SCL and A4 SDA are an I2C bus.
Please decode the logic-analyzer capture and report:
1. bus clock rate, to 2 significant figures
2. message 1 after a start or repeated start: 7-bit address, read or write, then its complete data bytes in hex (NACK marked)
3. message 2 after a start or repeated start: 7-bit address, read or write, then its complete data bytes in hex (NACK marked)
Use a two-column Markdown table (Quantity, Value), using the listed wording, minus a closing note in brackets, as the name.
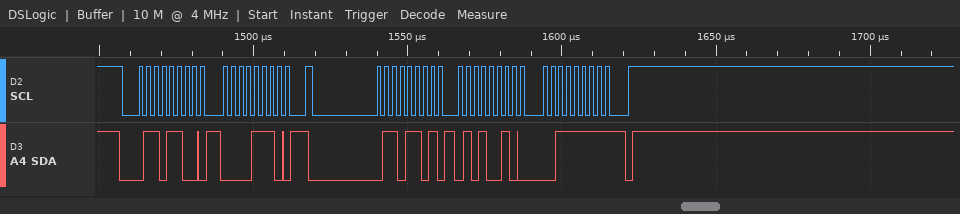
| Quantity | Value |
|---|---|
| bus clock rate, to 2 significant figures | 400 kHz |
| message 1 after a start or repeated start: 7-bit address, read or write, then its complete data bytes in hex | 0x36 write: 0E |
| message 2 after a start or repeated start: 7-bit address, read or write, then its complete data bytes in hex | 0x36 read: 52 3F NACK |
